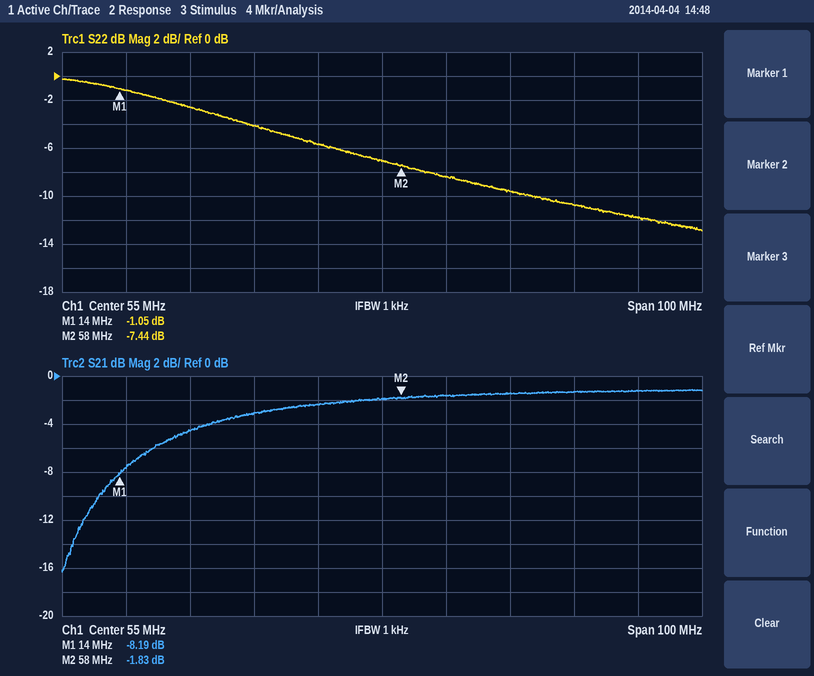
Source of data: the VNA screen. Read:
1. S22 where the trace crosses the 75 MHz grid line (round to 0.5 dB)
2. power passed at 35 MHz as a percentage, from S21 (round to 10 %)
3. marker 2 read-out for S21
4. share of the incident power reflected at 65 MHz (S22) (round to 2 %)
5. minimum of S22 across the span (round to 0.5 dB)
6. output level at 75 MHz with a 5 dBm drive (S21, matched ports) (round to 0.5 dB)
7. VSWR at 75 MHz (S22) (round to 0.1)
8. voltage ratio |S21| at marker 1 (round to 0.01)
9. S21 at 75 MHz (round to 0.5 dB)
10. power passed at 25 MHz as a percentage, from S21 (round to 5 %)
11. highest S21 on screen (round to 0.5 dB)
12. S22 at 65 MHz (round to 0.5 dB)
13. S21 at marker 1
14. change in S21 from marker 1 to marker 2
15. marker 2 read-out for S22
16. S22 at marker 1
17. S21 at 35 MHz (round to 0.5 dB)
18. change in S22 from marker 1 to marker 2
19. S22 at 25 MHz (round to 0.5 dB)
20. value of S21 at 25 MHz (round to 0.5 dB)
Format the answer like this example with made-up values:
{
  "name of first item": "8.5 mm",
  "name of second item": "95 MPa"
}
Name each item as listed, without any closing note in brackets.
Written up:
{
  "S22 where the trace crosses the 75 MHz grid line": "-9.5 dB",
  "power passed at 35 MHz as a percentage, from S21": "50 %",
  "marker 2 read-out for S21": "-1.83 dB",
  "share of the incident power reflected at 65 MHz (S22)": "14 %",
  "minimum of S22 across the span": "-13.0 dB",
  "output level at 75 MHz with a 5 dBm drive (S21, matched ports)": "3.5 dBm",
  "VSWR at 75 MHz (S22)": "2.0",
  "voltage ratio |S21| at marker 1": "0.39",
  "S21 at 75 MHz": "-1.5 dB",
  "power passed at 25 MHz as a percentage, from S21": "35 %",
  "highest S21 on screen": "-1.0 dB",
  "S22 at 65 MHz": "-8.5 dB",
  "S21 at marker 1": "-8.19 dB",
  "change in S21 from marker 1 to marker 2": "6.36 dB",
  "marker 2 read-out for S22": "-7.44 dB",
  "S22 at marker 1": "-1.05 dB",
  "S21 at 35 MHz": "-3.0 dB",
  "change in S22 from marker 1 to marker 2": "-6.39 dB",
  "S22 at 25 MHz": "-2.5 dB",
  "value of S21 at 25 MHz": "-4.5 dB"
}
